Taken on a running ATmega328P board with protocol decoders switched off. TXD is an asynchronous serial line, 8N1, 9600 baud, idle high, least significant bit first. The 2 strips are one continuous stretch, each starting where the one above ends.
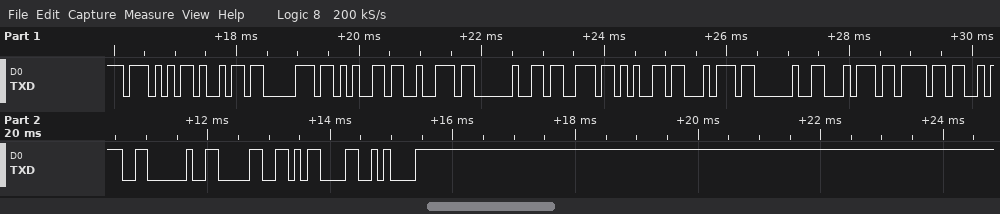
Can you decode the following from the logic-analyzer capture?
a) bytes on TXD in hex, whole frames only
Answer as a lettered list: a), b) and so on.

a) 0x57 0x69 0x70 0x65 0x72 0x20 0x73 0x65 0x74 0x20 0x74 0x6F 0x3A 0x20 0x30 0x0D 0x0A
